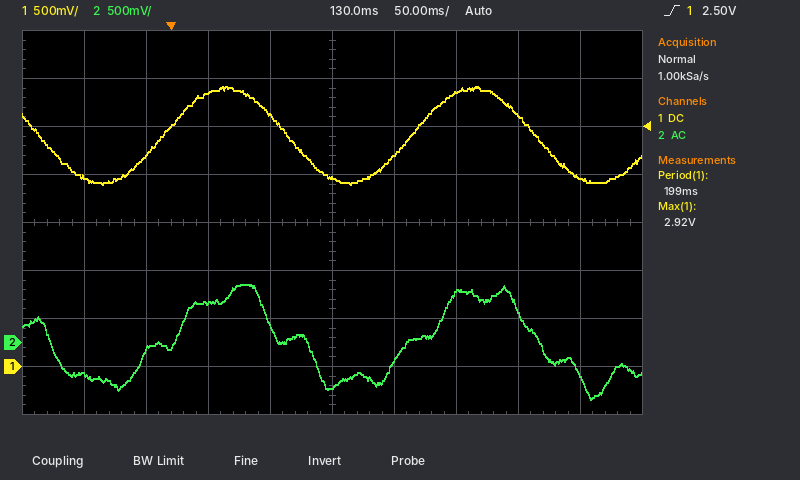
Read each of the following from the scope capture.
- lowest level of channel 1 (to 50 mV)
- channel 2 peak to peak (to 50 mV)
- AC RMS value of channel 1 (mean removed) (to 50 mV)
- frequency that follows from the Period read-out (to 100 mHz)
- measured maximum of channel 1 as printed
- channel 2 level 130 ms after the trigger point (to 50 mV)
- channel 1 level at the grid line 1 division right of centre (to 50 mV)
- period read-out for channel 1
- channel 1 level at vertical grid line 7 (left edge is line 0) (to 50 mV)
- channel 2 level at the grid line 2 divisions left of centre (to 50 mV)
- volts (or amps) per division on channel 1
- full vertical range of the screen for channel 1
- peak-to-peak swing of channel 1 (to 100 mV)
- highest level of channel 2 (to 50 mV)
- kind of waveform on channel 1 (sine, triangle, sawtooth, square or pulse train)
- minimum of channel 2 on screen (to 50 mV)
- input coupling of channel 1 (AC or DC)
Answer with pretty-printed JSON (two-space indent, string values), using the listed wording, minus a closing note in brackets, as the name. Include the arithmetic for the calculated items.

{
  "lowest level of channel 1": "1.90 V",
  "channel 2 peak to peak": "600 mV − (-600 mV) = 1.20 V",
  "AC RMS value of channel 1 (mean removed)": "1.00 V / (2√2) ≈ 354 mV, so 350 mV to the nearest 50 mV",
  "frequency that follows from the Period read-out": "1 / 199 ms ≈ 5.0 Hz",
  "measured maximum of channel 1 as printed": "2.92 V",
  "channel 2 level 130 ms after the trigger point": "-450 mV",
  "channel 1 level at the grid line 1 division right of centre": "2.20 V",
  "period read-out for channel 1": "199 ms",
  "channel 1 level at vertical grid line 7 (left edge is line 0)": "2.85 V",
  "channel 2 level at the grid line 2 divisions left of centre": "400 mV",
  "volts (or amps) per division on channel 1": "500 mV",
  "full vertical range of the screen for channel 1": "4 V",
  "peak-to-peak swing of channel 1": "1.00 V",
  "highest level of channel 2": "600 mV",
  "kind of waveform on channel 1": "sine",
  "minimum of channel 2 on screen": "-600 mV",
  "input coupling of channel 1": "DC"
}
